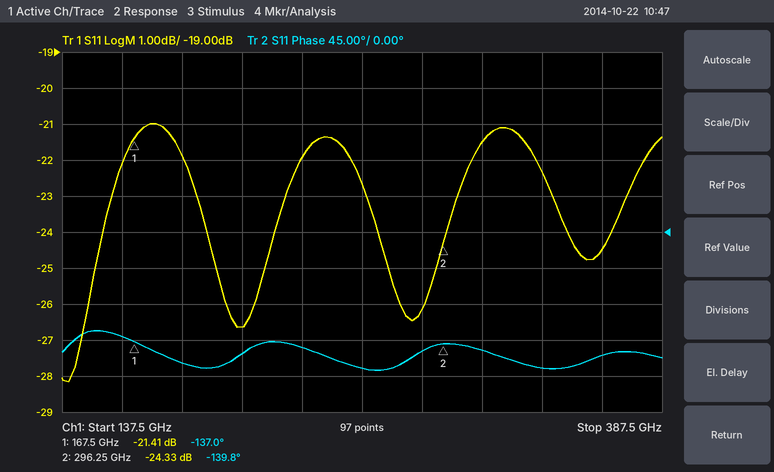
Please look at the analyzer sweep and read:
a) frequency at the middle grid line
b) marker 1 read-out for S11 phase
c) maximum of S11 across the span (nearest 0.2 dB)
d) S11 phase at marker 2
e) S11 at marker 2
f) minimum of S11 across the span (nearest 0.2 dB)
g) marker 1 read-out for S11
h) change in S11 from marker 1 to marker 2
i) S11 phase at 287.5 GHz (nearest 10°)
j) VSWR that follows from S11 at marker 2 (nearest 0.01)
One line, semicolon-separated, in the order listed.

262.5 GHz; -137.0°; -21.0 dB; -139.8°; -24.33 dB; -28.2 dB; -21.41 dB; -2.92 dB; -150°; 1.13
